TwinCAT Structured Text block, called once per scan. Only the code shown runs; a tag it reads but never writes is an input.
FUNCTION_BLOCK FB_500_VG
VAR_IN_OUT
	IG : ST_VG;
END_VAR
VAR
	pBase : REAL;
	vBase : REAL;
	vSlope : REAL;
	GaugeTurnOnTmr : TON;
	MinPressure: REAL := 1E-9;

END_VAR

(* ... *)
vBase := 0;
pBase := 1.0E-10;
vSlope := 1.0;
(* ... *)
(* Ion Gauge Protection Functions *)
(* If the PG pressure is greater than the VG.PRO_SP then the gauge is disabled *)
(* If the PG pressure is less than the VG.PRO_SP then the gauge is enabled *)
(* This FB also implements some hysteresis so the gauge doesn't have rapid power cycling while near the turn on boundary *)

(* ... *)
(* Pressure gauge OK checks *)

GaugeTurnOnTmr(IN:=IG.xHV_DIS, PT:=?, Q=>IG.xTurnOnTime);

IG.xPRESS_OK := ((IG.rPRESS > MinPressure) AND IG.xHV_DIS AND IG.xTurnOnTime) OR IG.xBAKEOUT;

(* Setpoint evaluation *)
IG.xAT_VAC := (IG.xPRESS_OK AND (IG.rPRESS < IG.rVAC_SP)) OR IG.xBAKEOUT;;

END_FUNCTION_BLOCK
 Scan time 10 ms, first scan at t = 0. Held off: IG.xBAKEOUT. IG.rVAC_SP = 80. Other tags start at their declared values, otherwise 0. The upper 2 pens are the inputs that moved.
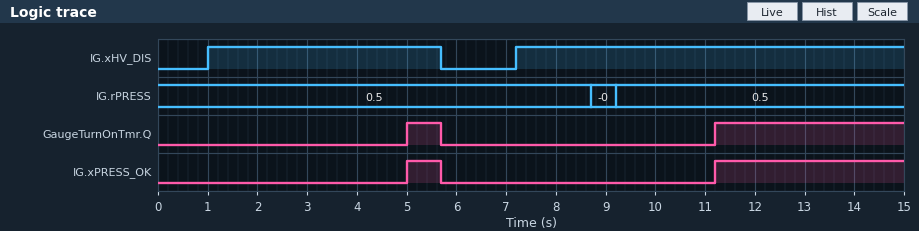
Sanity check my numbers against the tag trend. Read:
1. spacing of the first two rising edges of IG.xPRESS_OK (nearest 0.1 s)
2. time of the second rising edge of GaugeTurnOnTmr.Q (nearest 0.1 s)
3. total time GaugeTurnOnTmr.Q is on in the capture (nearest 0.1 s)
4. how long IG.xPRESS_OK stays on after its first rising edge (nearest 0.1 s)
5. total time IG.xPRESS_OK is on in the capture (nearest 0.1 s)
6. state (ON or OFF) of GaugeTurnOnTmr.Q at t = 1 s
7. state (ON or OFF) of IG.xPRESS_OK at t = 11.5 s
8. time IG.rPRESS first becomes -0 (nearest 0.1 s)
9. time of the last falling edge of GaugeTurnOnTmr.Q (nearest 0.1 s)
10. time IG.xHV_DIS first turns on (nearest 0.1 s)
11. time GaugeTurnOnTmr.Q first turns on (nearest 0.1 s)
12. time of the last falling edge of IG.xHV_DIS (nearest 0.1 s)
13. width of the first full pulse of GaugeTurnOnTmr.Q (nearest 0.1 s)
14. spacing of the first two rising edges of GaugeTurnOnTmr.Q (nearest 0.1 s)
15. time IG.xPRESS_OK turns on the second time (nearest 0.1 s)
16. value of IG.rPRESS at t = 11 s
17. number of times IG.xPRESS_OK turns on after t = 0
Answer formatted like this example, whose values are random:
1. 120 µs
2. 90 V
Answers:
1. 6.2 s
2. 11.2 s
3. 4.5 s
4. 0.7 s
5. 4.5 s
6. OFF
7. ON
8. 8.7 s
9. 5.7 s
10. 1.0 s
11. 5.0 s
12. 5.7 s
13. 0.7 s
14. 6.2 s
15. 11.2 s
16. 0.5
17. 2
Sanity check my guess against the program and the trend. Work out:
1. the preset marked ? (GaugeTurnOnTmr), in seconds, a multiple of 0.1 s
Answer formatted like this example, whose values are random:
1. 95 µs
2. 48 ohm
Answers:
1. 4.0 s
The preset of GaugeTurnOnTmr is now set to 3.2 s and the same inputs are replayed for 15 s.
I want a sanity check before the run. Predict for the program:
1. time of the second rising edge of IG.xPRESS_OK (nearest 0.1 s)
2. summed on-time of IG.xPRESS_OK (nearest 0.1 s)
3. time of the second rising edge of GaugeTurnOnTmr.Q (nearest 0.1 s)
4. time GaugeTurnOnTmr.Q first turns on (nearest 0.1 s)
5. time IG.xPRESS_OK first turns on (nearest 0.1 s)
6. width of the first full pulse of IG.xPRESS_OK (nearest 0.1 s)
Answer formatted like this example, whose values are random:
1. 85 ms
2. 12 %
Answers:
1. 10.4 s
2. 6.1 s
3. 10.4 s
4. 4.2 s
5. 4.2 s
6. 1.5 s
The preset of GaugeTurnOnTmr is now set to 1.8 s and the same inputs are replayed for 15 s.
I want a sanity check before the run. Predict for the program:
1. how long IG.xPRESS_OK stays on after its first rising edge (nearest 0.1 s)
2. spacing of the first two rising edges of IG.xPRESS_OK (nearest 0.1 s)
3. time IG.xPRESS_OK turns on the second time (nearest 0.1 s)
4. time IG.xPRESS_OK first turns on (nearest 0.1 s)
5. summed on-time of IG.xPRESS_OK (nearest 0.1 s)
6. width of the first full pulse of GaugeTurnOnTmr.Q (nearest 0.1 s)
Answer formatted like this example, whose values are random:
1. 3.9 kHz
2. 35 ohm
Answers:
1. 2.9 s
2. 6.4 s
3. 9.2 s
4. 2.8 s
5. 8.7 s
6. 2.9 s
